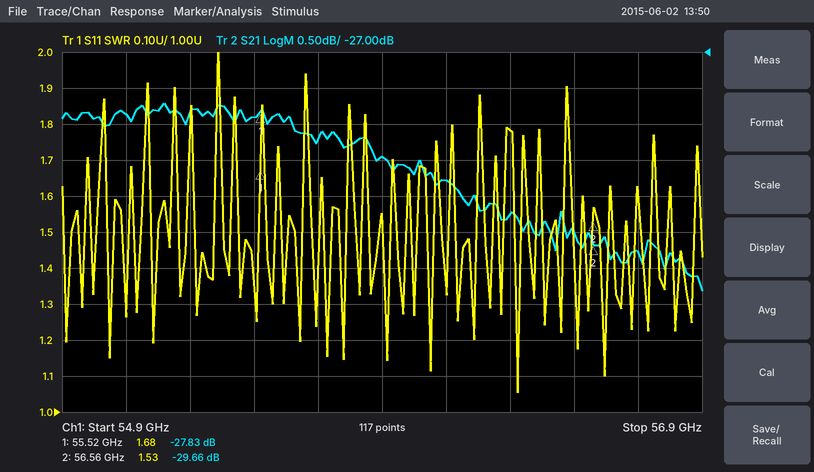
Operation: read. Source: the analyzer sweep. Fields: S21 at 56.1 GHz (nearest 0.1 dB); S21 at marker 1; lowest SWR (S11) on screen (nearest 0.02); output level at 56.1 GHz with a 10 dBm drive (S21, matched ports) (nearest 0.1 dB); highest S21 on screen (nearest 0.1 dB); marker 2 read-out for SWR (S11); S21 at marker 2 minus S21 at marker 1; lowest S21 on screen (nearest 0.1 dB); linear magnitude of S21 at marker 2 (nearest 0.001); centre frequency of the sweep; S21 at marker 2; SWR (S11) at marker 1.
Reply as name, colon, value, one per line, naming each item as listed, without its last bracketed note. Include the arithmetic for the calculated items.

S21 at 56.1 GHz: -28.8 dB
S21 at marker 1: -27.83 dB
lowest SWR (S11) on screen: 1.06
output level at 56.1 GHz with a 10 dBm drive (S21, matched ports): 10 dBm + (-28.8 dB) = -18.8 dBm
highest S21 on screen: -27.7 dB
marker 2 read-out for SWR: 1.53
S21 at marker 2 minus S21 at marker 1: -29.66 − (-27.83) = -1.83 dB
lowest S21 on screen: -30.3 dB
linear magnitude of S21 at marker 2: 10^(-29.66/20) ≈ 0.033
centre frequency of the sweep: 55.9 GHz
S21 at marker 2: -29.66 dB
SWR (S11) at marker 1: 1.68
